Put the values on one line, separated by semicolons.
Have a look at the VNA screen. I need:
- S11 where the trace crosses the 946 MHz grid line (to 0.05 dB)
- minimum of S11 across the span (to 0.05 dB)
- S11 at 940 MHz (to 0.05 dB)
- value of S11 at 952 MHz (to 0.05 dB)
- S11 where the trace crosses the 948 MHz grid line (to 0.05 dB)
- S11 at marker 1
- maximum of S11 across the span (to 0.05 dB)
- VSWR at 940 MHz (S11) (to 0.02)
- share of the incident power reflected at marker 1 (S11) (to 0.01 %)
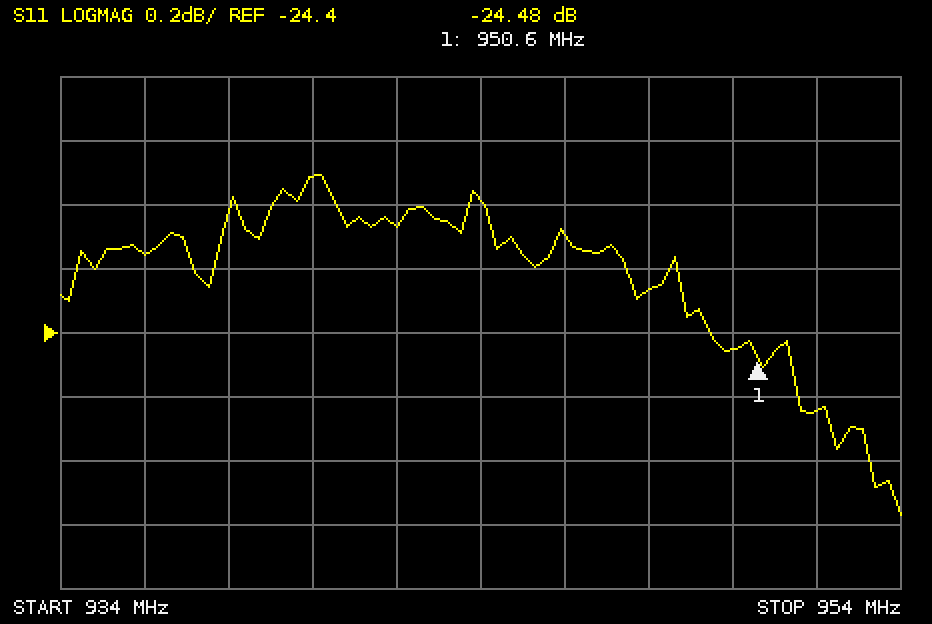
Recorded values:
-24.10 dB; -24.95 dB; -23.90 dB; -24.65 dB; -24.25 dB; -24.48 dB; -23.90 dB; 1.14; 0.36 %
